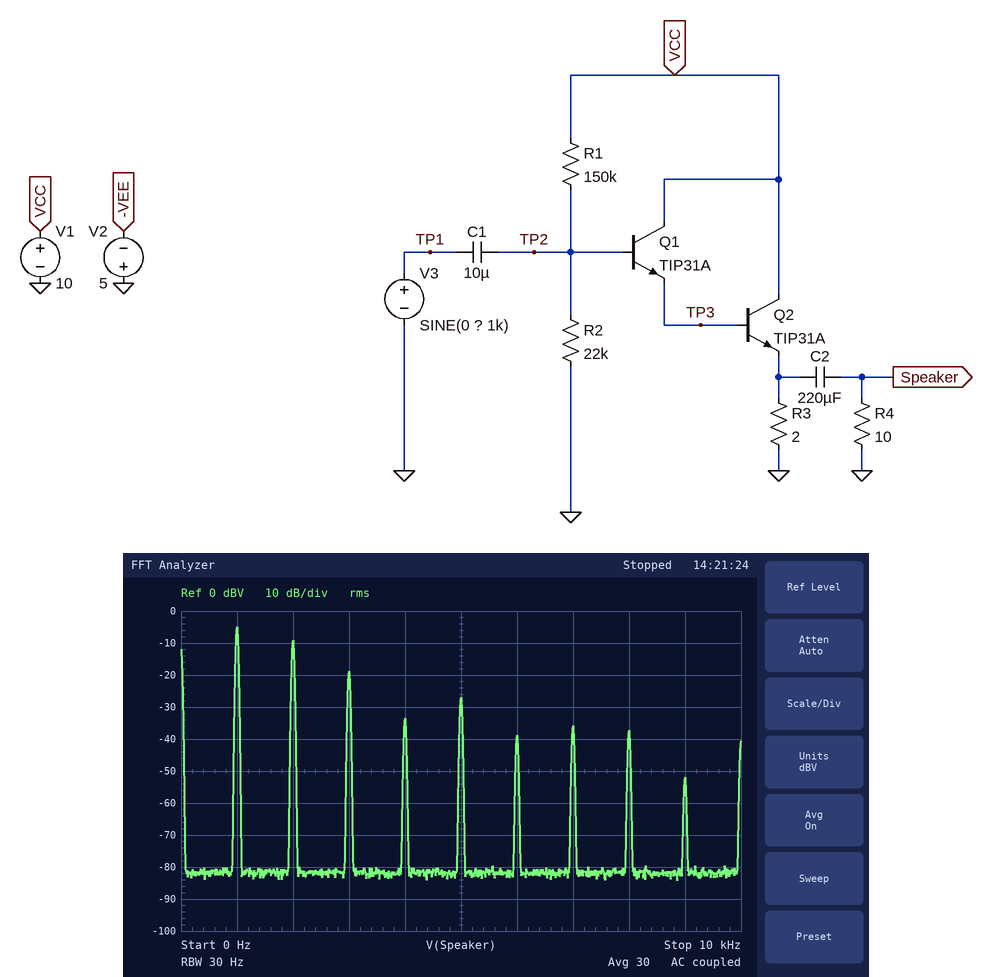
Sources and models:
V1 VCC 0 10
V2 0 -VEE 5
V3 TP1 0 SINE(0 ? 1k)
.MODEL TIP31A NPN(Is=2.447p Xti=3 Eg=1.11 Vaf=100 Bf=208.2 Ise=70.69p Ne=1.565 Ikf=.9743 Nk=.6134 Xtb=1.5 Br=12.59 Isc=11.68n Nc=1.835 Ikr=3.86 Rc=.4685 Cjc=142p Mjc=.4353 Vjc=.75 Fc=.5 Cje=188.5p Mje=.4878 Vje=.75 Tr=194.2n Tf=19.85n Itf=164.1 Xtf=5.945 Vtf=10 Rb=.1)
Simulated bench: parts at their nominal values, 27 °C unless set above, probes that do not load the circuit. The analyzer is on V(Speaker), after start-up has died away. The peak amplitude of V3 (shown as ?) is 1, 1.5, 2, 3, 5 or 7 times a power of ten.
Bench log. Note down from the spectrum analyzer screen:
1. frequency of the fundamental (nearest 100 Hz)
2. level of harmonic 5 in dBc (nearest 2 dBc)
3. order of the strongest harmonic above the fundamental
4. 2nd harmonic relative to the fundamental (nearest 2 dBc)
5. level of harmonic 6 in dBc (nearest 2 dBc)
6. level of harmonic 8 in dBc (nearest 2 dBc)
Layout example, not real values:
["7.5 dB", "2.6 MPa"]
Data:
["1.0 kHz", "-22 dBc", "2", "-4 dBc", "-34 dBc", "-32 dBc"]
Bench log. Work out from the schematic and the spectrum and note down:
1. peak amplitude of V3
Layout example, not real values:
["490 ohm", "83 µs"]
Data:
["3 V"]
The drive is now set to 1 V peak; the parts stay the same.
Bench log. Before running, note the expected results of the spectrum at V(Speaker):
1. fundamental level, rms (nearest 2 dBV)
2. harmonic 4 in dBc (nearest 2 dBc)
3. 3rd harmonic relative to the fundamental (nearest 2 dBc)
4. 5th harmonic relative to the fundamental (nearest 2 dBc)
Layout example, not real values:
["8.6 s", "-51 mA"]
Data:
["-14 dBV", "-24 dBc", "-18 dBc", "-26 dBc"]
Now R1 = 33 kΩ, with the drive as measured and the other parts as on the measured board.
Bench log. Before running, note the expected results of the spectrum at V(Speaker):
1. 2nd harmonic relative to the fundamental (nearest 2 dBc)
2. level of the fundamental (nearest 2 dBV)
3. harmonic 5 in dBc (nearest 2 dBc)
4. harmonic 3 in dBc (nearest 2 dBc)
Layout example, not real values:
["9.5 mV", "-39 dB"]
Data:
["-10 dBc", "2 dBV", "-32 dBc", "-26 dBc"]
